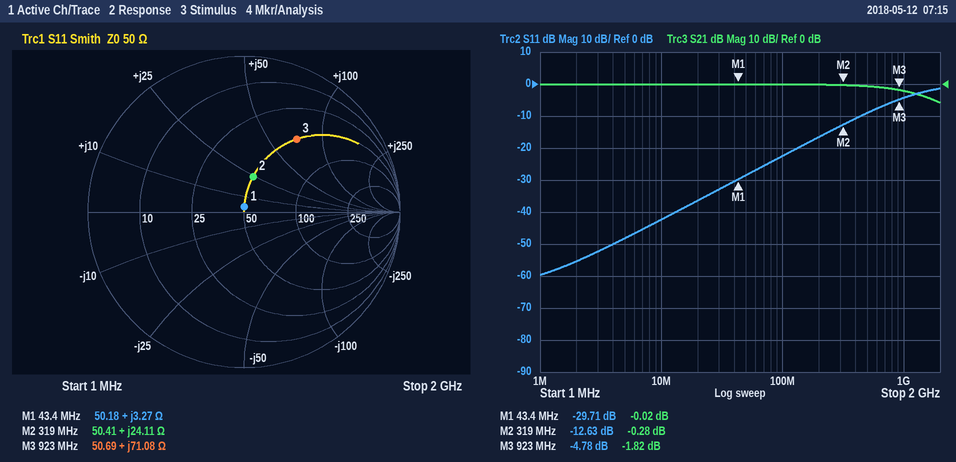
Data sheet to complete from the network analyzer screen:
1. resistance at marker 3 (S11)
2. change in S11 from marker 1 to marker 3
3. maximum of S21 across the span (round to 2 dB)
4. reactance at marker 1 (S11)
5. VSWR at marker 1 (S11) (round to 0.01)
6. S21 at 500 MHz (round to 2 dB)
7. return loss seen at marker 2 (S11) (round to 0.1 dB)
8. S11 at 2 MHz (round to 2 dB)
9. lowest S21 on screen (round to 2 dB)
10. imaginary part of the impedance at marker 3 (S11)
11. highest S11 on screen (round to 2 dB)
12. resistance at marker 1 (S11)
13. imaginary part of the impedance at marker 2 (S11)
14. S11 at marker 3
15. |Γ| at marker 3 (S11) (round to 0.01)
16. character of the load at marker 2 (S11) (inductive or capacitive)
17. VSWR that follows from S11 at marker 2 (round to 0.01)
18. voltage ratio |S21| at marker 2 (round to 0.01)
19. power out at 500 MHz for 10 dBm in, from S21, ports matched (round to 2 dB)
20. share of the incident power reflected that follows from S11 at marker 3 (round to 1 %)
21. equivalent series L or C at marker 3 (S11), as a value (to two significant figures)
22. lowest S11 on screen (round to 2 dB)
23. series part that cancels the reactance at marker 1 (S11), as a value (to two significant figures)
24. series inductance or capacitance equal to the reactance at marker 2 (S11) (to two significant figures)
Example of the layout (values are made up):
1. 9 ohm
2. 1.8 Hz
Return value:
1. 50.69 Ω
2. 24.93 dB
3. 0 dB
4. +3.27 Ω
5. 1.07
6. 0 dB
7. 12.6 dB
8. -56 dB
9. -6 dB
10. +71.08 Ω
11. -2 dB
12. 50.18 Ω
13. +24.11 Ω
14. -4.78 dB
15. 0.58
16. inductive
17. 1.61
18. 0.97
19. 10 dBm
20. 33 %
21. 12 nH
22. -60 dB
23. 1.1 nF
24. 12 nH
